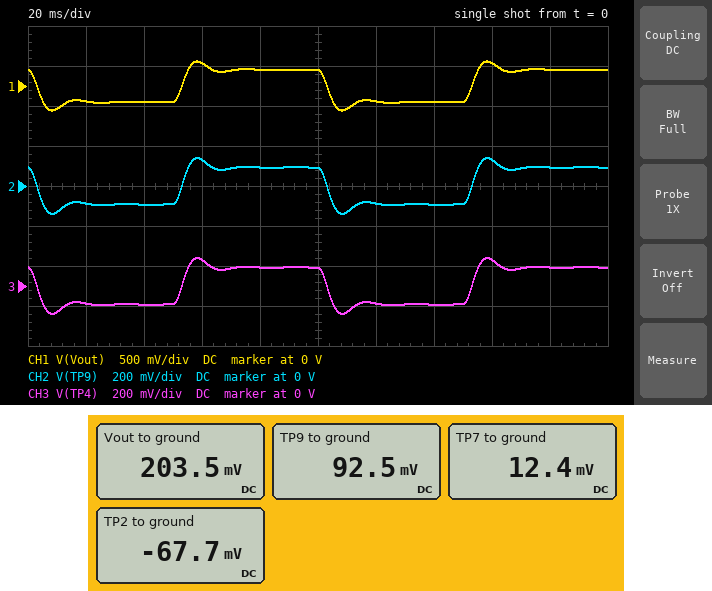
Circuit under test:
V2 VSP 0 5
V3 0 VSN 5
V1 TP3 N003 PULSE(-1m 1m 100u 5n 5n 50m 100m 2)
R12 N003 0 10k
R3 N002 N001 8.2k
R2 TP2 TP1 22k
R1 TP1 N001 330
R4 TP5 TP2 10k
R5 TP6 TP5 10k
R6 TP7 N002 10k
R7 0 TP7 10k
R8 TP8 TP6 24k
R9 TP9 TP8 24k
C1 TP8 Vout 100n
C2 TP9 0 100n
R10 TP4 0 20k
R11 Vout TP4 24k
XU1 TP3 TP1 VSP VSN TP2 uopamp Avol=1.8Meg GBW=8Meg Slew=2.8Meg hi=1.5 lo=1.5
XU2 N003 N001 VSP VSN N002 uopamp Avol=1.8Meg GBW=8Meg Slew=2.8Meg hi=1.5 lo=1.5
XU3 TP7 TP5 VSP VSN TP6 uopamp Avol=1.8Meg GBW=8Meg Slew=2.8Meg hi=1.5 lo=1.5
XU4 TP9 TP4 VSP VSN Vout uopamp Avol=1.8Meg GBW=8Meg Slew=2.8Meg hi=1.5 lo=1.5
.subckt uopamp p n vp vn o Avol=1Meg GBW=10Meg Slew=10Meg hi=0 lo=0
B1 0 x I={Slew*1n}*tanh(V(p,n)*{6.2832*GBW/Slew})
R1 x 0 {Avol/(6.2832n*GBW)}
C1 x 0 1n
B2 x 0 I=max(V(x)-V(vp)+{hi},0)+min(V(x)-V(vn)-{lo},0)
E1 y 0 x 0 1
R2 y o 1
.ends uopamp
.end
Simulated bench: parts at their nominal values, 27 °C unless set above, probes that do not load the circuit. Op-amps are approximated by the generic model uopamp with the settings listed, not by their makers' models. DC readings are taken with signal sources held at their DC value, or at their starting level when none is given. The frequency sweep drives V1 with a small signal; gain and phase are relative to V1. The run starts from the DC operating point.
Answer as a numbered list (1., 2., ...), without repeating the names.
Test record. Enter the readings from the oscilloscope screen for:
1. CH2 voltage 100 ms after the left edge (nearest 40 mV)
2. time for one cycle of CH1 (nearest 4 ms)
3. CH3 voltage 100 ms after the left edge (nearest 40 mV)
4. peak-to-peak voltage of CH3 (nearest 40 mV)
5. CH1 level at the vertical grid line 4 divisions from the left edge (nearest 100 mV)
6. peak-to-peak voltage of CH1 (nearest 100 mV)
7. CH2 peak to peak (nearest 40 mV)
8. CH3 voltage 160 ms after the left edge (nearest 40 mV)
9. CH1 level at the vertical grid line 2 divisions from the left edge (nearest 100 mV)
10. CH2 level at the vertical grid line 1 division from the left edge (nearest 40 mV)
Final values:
1. 80 mV
2. 100 ms
3. 80 mV
4. 280 mV
5. 200 mV
6. 600 mV
7. 280 mV
8. 120 mV
9. -200 mV
10. -80 mV
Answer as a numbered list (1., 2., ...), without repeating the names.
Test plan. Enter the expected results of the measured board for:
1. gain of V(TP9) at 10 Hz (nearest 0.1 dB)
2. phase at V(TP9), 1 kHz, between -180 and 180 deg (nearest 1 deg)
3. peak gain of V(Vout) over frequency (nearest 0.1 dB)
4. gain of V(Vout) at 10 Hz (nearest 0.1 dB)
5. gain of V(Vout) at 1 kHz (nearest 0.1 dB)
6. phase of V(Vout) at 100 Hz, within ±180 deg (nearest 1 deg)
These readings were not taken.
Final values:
1. 39.5 dB
2. 2 deg
3. 48.9 dB
4. 46.3 dB
5. -0.9 dB
6. 43 deg
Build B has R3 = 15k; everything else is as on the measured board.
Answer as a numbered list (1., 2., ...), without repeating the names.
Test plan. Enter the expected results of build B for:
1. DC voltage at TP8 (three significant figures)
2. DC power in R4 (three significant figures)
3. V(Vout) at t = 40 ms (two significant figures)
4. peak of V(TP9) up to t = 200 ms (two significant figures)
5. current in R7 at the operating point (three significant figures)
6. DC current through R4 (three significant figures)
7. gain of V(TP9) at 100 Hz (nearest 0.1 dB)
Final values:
1. 113 mV
2. 817 nW
3. -250 mV
4. 170 mV
5. 2.27 µA
6. 9.04 µA
7. 36.2 dB
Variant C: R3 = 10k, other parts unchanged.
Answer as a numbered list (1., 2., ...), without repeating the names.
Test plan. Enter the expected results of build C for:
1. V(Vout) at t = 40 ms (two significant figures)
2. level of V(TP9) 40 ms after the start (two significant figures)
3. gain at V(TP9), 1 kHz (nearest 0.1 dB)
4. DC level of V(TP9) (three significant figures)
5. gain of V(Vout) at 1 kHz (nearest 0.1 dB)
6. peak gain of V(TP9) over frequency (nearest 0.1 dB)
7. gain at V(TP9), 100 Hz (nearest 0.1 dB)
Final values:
1. -220 mV
2. -98 mV
3. -7.3 dB
4. 98.0 mV
5. -0.4 dB
6. 42.5 dB
7. 34.9 dB
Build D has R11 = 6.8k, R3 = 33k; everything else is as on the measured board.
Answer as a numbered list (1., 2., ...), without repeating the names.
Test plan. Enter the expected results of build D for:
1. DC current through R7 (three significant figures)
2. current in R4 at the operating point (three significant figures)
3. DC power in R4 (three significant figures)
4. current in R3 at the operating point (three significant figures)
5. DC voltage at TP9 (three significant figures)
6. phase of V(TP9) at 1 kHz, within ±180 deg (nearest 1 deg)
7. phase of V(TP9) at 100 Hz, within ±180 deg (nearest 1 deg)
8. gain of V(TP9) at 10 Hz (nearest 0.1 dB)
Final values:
1. 5.00 µA
2. 11.8 µA
3. 1.38 µW
4. 3.03 µA
5. 168 mV
6. 5 deg
7. 63 deg
8. 44.4 dB
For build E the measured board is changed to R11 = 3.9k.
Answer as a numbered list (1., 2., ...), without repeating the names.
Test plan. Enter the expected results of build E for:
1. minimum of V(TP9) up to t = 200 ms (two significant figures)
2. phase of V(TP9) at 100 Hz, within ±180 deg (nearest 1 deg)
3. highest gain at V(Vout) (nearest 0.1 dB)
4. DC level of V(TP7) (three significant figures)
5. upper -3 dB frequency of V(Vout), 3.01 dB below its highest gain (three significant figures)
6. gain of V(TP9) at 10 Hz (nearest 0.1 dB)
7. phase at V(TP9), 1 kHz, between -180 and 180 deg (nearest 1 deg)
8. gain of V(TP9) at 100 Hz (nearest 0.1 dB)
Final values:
1. -93 mV
2. 65 deg
3. 40.9 dB
4. 12.4 mV
5. 49.3 Hz
6. 39.2 dB
7. 6 deg
8. 29.8 dB
